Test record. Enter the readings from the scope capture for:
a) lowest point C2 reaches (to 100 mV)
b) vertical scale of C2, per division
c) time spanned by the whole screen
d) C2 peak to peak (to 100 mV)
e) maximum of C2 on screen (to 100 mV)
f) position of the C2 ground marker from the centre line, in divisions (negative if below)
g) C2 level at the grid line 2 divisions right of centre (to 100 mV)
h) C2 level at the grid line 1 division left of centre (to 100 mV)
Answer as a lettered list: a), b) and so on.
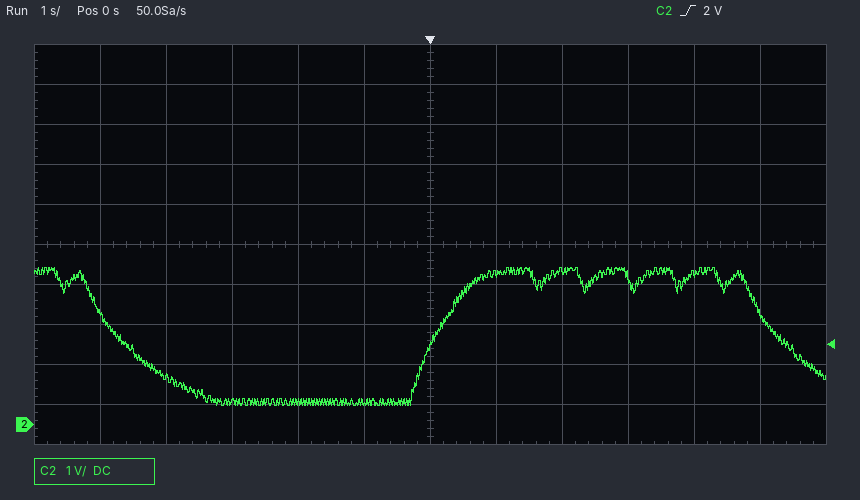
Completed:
a) 500 mV
b) 1 V
c) 12 s
d) 3.4 V
e) 3.9 V
f) -4.5 div
g) 3.8 V
h) 600 mV
